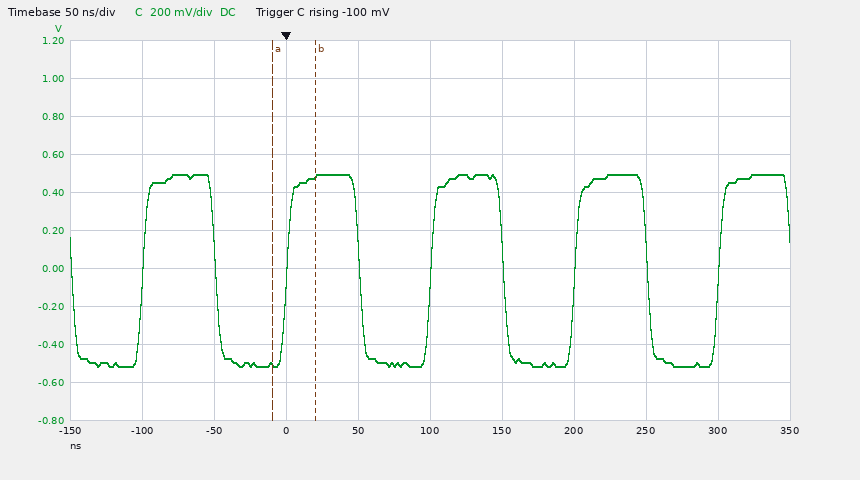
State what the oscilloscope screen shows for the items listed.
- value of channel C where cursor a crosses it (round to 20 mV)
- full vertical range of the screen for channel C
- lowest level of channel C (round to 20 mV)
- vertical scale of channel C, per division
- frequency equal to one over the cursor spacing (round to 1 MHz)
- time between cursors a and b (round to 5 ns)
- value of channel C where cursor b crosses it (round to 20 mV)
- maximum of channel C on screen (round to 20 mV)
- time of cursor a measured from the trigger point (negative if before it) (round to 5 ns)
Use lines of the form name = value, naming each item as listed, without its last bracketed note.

value of channel C where cursor a crosses it = -500 mV
full vertical range of the screen for channel C = 2 V
lowest level of channel C = -520 mV
vertical scale of channel C, per division = 200 mV
frequency equal to one over the cursor spacing = 33 MHz
time between cursors a and b = 30 ns
value of channel C where cursor b crosses it = 480 mV
maximum of channel C on screen = 500 mV
time of cursor a measured from the trigger point (negative if before it) = -10 ns
